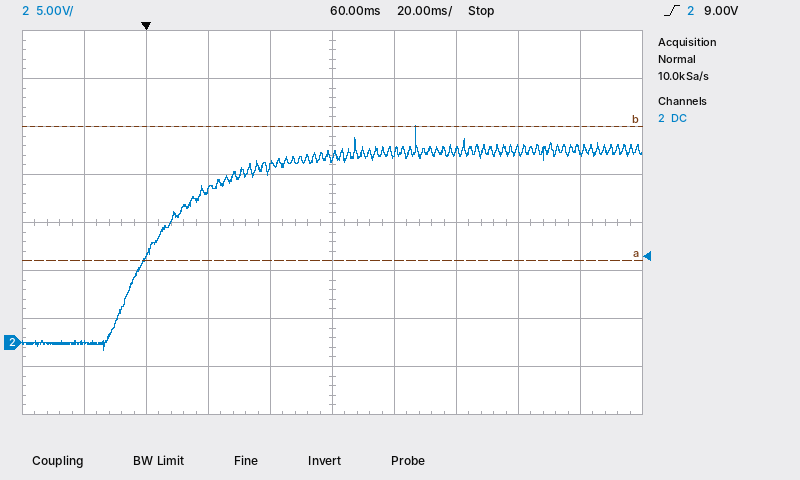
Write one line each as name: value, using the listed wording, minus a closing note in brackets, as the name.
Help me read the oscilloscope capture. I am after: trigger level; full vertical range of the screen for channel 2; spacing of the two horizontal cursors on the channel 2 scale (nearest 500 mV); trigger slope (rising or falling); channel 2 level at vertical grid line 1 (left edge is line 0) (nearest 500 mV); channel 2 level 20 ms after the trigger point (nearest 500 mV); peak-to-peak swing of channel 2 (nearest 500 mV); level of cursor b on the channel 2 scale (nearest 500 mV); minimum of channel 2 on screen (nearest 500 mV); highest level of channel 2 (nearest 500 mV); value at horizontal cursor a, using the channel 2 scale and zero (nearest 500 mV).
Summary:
trigger level: 9.00 V
full vertical range of the screen for channel 2: 40 V
spacing of the two horizontal cursors on the channel 2 scale: 14.0 V
trigger slope: rising
channel 2 level at vertical grid line 1 (left edge is line 0): 0.0 V
channel 2 level 20 ms after the trigger point: 16.0 V
peak-to-peak swing of channel 2: 23.5 V
level of cursor b on the channel 2 scale: 22.5 V
minimum of channel 2 on screen: -1.0 V
highest level of channel 2: 22.5 V
value at horizontal cursor a, using the channel 2 scale and zero: 8.5 V
